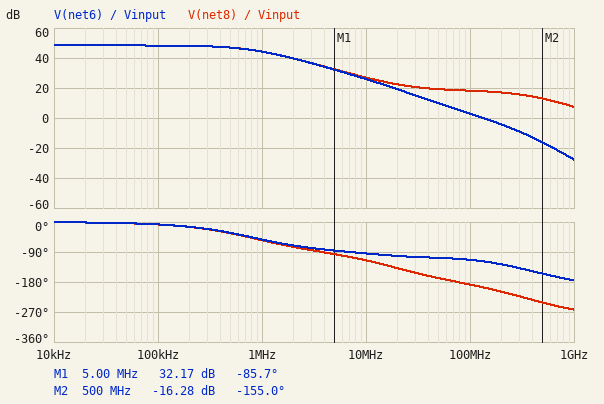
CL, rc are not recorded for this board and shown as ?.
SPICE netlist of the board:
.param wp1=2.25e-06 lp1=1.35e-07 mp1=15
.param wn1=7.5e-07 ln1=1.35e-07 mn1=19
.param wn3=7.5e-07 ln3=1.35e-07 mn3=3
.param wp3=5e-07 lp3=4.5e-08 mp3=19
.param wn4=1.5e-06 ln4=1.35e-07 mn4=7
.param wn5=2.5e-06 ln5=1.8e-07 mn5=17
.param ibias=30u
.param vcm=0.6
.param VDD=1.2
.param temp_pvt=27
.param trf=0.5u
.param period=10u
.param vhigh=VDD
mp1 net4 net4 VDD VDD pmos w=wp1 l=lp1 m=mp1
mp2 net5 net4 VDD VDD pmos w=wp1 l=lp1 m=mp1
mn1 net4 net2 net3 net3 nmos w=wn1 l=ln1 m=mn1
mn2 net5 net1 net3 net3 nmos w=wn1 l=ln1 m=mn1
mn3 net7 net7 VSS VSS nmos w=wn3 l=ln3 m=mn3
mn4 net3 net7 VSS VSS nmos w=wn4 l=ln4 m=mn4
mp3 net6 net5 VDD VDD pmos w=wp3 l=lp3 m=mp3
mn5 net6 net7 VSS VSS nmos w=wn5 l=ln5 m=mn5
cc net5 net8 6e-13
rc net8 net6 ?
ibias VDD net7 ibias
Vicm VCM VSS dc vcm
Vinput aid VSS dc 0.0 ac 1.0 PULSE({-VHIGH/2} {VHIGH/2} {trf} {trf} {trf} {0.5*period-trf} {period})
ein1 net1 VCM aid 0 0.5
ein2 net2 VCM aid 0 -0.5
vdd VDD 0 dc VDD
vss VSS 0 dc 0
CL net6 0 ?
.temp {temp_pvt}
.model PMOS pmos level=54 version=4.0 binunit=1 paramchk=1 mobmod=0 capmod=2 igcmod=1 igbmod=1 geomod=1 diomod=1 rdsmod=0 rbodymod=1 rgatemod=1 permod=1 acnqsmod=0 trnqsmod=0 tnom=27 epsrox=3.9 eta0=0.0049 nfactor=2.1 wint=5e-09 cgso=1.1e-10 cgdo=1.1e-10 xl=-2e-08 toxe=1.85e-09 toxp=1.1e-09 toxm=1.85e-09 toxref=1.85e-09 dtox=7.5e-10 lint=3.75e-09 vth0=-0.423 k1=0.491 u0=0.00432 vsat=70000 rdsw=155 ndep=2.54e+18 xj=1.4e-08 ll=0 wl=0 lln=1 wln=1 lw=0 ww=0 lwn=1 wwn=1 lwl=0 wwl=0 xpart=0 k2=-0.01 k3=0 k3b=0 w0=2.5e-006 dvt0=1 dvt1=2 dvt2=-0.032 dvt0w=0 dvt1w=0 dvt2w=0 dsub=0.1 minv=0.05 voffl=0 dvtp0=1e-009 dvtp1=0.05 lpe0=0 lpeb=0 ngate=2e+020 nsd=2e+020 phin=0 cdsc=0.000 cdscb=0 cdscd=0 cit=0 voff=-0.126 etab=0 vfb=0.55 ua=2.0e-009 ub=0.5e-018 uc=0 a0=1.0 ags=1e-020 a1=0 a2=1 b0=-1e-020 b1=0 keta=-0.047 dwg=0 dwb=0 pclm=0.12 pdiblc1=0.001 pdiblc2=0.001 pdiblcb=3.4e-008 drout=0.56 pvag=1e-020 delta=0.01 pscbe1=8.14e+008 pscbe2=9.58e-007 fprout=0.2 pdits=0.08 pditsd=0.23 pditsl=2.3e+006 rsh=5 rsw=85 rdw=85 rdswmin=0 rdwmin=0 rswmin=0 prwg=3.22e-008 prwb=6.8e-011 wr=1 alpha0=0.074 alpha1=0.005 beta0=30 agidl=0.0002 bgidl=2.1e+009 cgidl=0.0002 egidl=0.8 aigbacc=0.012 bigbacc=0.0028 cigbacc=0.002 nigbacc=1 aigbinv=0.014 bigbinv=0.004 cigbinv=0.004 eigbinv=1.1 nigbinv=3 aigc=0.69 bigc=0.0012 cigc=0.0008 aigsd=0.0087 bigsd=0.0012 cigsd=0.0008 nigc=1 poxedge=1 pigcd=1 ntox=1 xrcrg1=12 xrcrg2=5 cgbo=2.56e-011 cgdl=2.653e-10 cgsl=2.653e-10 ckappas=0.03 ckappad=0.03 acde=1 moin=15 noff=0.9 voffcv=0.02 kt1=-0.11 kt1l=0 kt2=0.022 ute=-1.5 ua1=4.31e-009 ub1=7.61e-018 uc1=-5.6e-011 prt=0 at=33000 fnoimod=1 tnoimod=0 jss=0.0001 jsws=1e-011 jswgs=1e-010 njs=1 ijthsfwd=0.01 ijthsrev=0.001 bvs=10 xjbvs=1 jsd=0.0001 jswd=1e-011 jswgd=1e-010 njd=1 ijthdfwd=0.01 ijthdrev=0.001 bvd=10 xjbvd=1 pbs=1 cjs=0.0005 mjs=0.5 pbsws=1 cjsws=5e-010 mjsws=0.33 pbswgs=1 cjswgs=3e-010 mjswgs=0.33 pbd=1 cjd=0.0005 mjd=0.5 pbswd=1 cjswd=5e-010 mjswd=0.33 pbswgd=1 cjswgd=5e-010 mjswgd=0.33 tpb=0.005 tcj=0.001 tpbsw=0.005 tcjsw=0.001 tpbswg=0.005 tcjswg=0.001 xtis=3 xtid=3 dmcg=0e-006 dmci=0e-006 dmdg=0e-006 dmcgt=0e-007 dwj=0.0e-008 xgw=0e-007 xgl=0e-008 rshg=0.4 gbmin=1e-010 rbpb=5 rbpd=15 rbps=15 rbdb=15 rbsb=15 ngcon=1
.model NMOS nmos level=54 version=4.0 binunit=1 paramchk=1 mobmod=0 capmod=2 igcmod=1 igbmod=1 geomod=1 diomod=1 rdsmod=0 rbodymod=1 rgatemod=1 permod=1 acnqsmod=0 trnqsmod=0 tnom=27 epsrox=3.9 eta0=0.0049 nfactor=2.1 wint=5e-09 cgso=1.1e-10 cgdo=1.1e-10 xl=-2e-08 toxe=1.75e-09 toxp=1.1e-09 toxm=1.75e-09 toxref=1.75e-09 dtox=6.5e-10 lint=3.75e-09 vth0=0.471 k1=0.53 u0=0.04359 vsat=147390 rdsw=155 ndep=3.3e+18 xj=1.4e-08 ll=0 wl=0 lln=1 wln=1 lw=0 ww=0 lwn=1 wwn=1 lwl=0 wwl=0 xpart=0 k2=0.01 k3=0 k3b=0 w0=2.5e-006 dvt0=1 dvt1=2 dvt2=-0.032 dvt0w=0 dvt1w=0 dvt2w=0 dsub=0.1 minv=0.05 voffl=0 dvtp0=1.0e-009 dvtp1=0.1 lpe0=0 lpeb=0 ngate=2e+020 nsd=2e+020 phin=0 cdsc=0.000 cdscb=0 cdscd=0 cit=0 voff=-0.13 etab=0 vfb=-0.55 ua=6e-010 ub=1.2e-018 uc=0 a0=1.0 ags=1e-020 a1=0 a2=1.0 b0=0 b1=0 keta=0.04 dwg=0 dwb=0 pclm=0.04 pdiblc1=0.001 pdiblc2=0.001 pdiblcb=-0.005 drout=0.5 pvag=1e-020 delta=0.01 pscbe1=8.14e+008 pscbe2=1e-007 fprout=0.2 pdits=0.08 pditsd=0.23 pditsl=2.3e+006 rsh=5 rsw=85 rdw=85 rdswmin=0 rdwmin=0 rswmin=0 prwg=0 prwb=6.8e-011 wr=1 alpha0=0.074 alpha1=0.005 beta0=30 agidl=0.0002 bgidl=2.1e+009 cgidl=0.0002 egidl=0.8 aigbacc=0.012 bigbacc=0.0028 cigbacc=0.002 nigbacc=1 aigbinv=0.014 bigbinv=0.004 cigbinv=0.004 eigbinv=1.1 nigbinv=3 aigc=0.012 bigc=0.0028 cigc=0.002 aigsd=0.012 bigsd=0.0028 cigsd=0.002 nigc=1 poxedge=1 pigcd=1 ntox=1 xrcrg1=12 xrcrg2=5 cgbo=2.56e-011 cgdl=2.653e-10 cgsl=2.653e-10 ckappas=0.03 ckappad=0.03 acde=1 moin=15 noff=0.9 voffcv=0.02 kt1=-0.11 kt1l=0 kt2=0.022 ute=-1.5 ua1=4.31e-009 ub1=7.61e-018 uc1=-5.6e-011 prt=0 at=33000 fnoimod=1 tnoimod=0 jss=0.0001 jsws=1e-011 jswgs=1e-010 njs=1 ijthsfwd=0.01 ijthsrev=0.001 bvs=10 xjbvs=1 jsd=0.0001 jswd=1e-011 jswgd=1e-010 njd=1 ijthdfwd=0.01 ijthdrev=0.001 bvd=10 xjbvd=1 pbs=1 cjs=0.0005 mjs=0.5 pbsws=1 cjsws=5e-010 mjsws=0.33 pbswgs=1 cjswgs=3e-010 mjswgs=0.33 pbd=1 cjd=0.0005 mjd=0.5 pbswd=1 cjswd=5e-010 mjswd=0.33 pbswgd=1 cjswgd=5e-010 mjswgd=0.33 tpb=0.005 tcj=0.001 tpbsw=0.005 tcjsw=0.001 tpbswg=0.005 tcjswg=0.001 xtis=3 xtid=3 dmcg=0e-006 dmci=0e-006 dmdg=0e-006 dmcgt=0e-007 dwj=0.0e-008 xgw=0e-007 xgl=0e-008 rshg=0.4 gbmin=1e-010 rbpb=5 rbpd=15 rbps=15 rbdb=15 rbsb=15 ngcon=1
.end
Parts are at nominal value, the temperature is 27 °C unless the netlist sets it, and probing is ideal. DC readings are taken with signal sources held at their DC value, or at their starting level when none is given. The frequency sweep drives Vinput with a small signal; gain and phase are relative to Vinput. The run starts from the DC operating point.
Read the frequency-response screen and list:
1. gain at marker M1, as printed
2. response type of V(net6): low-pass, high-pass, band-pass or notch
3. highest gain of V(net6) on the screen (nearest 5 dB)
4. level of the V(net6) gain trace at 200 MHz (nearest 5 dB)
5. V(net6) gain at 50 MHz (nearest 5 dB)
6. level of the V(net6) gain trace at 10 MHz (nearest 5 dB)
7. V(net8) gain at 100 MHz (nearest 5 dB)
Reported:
32.17 dB
low-pass
50 dB
-5 dB
10 dB
25 dB
20 dB
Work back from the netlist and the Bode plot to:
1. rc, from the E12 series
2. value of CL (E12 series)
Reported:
8.2 kΩ
33 pF
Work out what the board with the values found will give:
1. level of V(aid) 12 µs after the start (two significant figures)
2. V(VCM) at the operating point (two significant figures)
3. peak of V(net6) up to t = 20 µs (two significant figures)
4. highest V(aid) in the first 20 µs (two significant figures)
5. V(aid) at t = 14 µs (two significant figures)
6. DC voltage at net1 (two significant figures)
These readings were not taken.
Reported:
600 mV
600 mV
1.2 V
600 mV
600 mV
600 mV
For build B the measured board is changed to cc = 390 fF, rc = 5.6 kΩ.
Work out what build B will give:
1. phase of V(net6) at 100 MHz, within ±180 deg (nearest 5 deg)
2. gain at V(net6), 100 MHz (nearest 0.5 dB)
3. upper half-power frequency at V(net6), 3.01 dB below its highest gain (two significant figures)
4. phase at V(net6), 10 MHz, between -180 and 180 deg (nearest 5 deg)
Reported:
-125 deg
1.0 dB
1.1 MHz
-100 deg
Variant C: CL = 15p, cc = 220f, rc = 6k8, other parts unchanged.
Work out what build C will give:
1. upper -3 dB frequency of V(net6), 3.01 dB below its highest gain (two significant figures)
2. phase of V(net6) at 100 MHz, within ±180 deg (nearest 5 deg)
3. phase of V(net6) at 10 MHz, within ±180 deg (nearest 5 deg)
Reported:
2.0 MHz
-125 deg
-85 deg
